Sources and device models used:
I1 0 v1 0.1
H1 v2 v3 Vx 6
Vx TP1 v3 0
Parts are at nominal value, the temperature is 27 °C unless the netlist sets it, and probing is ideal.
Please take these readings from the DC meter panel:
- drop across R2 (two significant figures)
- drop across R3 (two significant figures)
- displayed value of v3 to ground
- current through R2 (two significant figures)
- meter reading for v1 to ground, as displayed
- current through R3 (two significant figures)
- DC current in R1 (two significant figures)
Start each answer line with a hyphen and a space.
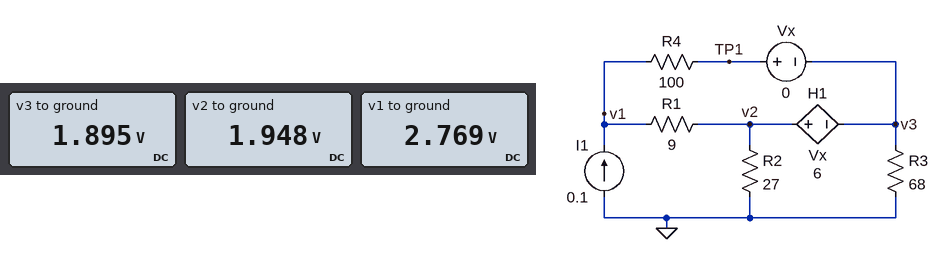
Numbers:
- 1.9 V
- 1.9 V
- 1.895 V
- 72 mA
- 2.769 V
- 28 mA
- 91 mA
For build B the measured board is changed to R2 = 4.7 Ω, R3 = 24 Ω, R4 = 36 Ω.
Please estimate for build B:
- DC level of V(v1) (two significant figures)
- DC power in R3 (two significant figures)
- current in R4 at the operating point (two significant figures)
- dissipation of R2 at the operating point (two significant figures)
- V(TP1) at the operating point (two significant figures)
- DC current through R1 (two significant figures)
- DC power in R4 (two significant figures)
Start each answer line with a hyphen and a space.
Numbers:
- 1.1 V
- 3.2 mW
- 23 mA
- 37 mW
- 280 mV
- 77 mA
- 19 mW
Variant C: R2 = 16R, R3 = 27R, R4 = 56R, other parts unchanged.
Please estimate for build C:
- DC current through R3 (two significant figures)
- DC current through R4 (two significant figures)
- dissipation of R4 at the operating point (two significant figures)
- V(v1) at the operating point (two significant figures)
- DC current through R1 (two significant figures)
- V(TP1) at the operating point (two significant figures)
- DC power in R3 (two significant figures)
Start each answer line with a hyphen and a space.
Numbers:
- 35 mA
- 15 mA
- 13 mW
- 1.8 V
- 85 mA
- 950 mV
- 33 mW
